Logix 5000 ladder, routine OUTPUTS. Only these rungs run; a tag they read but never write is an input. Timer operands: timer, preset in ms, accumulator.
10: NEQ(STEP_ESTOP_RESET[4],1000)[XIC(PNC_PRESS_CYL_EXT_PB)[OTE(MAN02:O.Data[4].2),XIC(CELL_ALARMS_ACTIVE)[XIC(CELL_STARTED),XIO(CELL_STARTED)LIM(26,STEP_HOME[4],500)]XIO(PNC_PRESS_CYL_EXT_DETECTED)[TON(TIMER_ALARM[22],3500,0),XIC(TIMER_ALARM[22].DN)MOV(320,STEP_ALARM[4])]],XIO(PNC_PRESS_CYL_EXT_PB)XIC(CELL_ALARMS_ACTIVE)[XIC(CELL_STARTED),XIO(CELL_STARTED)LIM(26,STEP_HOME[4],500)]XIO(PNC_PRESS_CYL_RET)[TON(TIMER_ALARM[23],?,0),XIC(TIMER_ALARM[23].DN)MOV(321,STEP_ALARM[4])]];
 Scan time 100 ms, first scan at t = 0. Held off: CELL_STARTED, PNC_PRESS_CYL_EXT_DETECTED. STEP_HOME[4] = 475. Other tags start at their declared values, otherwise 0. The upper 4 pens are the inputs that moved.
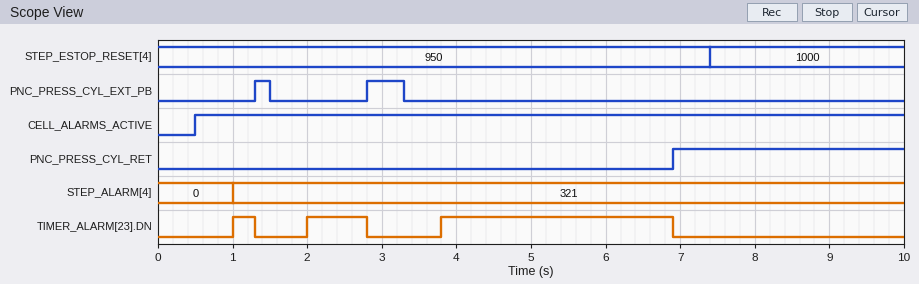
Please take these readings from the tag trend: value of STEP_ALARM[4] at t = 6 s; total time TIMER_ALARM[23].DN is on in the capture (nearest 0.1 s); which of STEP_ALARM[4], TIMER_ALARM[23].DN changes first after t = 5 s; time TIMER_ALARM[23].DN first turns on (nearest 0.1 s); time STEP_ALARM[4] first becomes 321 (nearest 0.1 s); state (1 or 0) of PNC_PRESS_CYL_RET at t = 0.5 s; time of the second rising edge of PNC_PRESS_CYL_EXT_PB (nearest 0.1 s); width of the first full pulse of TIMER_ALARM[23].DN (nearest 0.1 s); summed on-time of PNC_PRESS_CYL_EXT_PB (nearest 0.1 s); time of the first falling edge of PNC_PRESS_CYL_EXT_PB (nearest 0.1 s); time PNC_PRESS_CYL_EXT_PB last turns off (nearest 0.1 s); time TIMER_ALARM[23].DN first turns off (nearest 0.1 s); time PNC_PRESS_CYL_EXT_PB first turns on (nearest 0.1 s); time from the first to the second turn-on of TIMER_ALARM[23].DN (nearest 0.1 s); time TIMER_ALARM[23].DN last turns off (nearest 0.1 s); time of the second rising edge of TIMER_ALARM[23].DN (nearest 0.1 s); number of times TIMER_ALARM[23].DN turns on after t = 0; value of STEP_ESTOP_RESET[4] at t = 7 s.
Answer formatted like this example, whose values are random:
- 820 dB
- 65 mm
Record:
- 321
- 4.2 s
- TIMER_ALARM[23].DN
- 1.0 s
- 1.0 s
- 0
- 2.8 s
- 0.3 s
- 0.7 s
- 1.5 s
- 3.3 s
- 1.3 s
- 1.3 s
- 1.0 s
- 6.9 s
- 2.0 s
- 3
- 950
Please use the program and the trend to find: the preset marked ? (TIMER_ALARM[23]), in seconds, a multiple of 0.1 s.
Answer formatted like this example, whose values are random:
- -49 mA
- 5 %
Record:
- 0.5 s
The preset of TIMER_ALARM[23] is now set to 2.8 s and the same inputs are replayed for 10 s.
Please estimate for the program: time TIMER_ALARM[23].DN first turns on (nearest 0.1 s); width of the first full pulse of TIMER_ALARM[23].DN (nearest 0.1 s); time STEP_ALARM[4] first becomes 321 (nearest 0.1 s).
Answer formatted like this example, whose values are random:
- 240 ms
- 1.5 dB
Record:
- 6.1 s
- 0.8 s
- 6.1 s
